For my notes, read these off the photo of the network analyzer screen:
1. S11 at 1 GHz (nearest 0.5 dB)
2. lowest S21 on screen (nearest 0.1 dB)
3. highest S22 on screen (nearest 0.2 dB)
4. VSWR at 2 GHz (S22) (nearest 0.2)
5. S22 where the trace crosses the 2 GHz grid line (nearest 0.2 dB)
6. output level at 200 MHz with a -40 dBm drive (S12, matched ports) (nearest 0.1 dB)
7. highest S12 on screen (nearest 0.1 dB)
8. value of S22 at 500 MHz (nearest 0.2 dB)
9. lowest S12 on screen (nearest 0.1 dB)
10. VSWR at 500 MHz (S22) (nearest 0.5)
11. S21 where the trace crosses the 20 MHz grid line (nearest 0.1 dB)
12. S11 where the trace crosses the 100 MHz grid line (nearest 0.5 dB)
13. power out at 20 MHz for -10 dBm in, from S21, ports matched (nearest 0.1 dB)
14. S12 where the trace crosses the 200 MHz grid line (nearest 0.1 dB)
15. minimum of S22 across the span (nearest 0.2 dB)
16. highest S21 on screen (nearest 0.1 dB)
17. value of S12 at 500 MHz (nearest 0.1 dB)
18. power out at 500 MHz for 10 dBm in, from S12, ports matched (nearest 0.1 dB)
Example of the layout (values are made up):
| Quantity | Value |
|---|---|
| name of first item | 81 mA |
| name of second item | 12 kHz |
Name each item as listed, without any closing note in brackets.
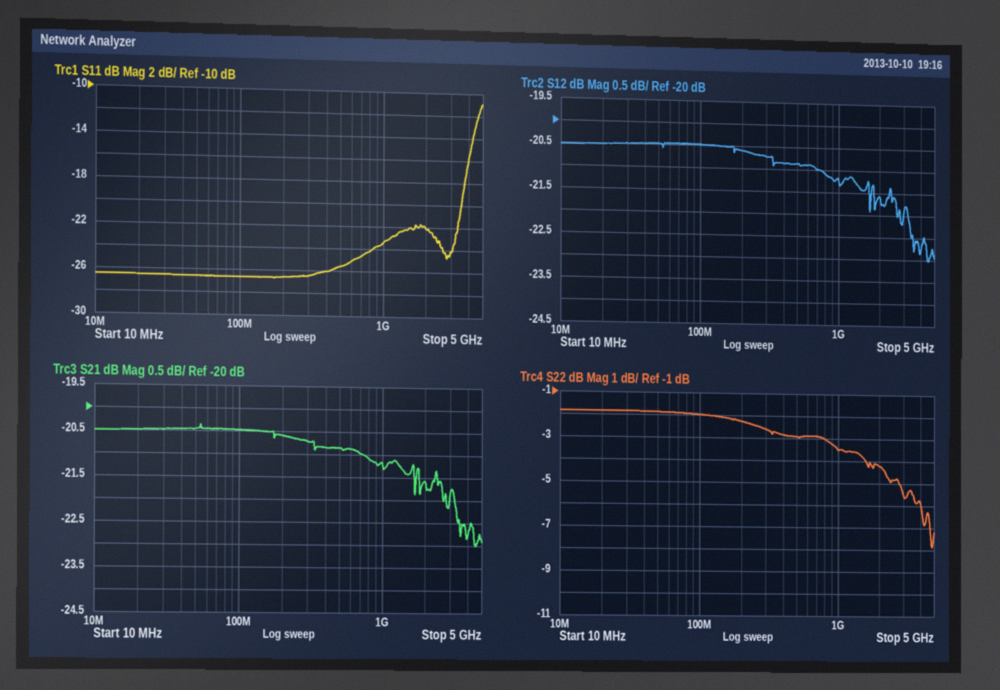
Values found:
| Quantity | Value |
|---|---|
| S11 at 1 GHz | -23.5 dB |
| lowest S21 on screen | -23.0 dB |
| highest S22 on screen | -1.8 dB |
| VSWR at 2 GHz (S22) | 4.2 |
| S22 where the trace crosses the 2 GHz grid line | -4.2 dB |
| output level at 200 MHz with a -40 dBm drive (S12, matched ports) | -60.6 dBm |
| highest S12 on screen | -20.5 dB |
| value of S22 at 500 MHz | -3.0 dB |
| lowest S12 on screen | -23.0 dB |
| VSWR at 500 MHz (S22) | 6.0 |
| S21 where the trace crosses the 20 MHz grid line | -20.5 dB |
| S11 where the trace crosses the 100 MHz grid line | -26.5 dB |
| power out at 20 MHz for -10 dBm in, from S21, ports matched | -30.5 dBm |
| S12 where the trace crosses the 200 MHz grid line | -20.6 dB |
| minimum of S22 across the span | -7.8 dB |
| highest S21 on screen | -20.4 dB |
| value of S12 at 500 MHz | -20.9 dB |
| power out at 500 MHz for 10 dBm in, from S12, ports matched | -10.9 dBm |
